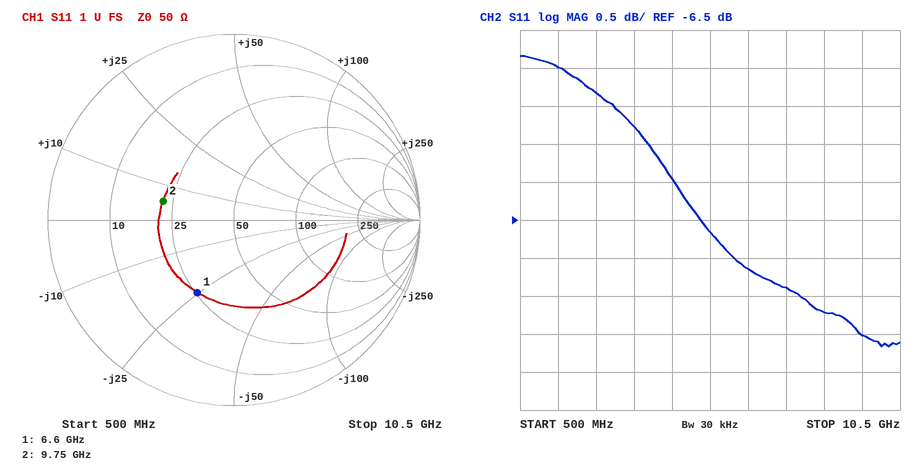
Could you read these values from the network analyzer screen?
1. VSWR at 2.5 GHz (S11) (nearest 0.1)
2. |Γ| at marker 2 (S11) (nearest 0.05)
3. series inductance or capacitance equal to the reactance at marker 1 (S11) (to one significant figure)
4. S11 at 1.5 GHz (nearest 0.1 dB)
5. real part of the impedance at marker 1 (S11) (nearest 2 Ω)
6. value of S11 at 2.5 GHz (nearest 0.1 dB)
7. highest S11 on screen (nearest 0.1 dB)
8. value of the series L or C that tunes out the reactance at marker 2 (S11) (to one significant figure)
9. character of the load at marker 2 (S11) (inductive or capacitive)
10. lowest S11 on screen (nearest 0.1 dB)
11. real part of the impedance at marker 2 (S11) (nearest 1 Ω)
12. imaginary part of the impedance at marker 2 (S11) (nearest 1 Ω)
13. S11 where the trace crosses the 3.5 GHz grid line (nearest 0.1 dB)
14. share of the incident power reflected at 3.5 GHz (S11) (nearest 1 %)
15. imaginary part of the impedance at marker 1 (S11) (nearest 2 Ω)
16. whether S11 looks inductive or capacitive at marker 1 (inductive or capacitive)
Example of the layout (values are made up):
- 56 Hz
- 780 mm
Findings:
- 3.7
- 0.40
- 1.0 pF
- -4.5 dB
- 26 Ω
- -4.8 dB
- -4.3 dB
- 3 pF
- inductive
- -8.2 dB
- 22 Ω
- +5 Ω
- -5.3 dB
- 30 %
- -24 Ω
- capacitive
